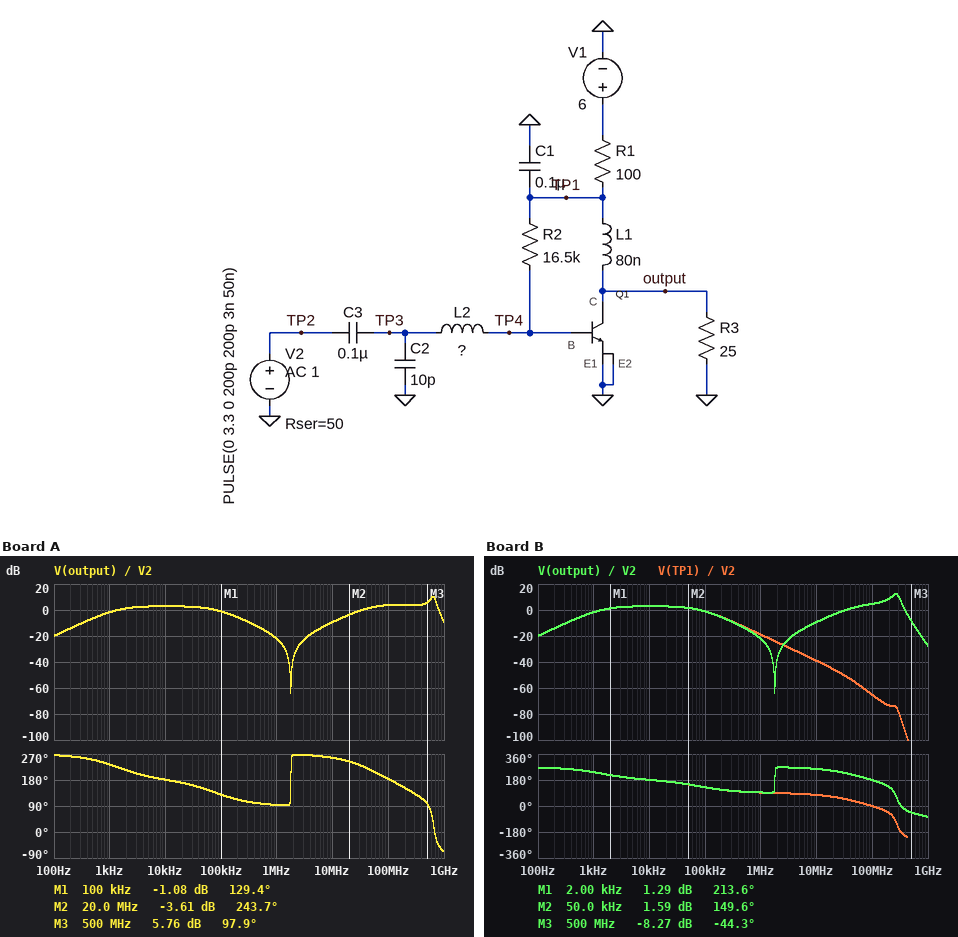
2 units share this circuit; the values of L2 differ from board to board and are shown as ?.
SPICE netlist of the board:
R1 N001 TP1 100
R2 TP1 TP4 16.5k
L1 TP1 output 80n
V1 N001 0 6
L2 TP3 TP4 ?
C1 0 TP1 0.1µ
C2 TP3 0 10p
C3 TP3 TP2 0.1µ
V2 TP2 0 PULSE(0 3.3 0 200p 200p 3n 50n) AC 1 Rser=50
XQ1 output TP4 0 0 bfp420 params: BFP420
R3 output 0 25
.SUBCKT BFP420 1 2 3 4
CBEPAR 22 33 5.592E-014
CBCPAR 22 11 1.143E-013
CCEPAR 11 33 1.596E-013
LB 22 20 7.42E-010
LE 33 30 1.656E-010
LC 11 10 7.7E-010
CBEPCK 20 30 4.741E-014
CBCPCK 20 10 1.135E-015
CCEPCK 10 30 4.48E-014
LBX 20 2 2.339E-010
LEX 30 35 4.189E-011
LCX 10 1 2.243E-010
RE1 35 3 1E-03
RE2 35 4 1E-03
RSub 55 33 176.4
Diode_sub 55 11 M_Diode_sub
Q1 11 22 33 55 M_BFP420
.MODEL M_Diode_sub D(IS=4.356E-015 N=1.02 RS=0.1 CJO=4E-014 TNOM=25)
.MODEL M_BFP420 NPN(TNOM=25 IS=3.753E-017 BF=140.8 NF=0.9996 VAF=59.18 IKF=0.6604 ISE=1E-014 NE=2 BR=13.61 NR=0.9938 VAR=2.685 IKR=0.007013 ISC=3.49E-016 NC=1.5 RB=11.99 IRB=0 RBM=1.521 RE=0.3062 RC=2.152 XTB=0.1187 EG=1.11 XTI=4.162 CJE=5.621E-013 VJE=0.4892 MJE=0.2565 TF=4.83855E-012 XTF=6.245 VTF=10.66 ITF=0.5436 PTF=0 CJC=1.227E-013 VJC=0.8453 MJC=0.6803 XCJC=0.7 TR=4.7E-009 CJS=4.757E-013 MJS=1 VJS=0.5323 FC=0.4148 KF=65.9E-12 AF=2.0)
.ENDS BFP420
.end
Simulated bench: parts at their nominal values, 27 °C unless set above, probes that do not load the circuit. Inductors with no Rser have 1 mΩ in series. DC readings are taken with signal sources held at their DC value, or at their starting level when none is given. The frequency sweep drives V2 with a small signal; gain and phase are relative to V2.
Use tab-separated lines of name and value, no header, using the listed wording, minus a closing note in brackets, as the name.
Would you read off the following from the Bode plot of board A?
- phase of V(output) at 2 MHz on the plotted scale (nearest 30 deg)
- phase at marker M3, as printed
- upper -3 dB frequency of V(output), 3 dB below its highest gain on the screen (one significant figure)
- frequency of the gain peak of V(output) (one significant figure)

phase of V(output) at 2 MHz on the plotted scale	270 deg
phase at marker M3, as printed	97.9 deg
upper -3 dB frequency of V(output), 3 dB below its highest gain on the screen	700 MHz
frequency of the gain peak of V(output)	600 MHz
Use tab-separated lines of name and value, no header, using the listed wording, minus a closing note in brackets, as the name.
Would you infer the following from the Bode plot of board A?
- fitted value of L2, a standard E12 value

fitted value of L2, a standard E12 value	33 nH
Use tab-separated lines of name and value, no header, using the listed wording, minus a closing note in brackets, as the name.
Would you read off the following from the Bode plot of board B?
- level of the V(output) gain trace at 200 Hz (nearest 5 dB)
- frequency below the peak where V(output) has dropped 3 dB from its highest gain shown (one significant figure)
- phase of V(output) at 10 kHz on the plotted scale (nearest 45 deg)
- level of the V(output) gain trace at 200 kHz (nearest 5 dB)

level of the V(output) gain trace at 200 Hz	-15 dB
frequency below the peak where V(output) has dropped 3 dB from its highest gain shown	200 MHz
phase of V(output) at 10 kHz on the plotted scale	180 deg
level of the V(output) gain trace at 200 kHz	-5 dB
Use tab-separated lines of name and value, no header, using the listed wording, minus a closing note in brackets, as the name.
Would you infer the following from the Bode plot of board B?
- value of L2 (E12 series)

value of L2	180 nH
